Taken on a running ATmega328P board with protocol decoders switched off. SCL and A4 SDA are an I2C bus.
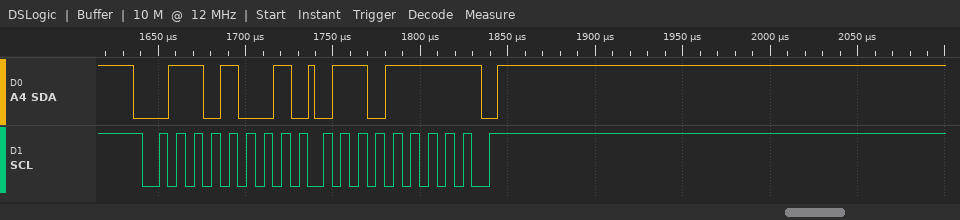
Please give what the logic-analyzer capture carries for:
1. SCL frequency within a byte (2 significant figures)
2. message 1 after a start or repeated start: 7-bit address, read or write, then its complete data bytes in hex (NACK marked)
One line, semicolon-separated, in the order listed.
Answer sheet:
100 kHz; 0x34 read: 6F NACK
